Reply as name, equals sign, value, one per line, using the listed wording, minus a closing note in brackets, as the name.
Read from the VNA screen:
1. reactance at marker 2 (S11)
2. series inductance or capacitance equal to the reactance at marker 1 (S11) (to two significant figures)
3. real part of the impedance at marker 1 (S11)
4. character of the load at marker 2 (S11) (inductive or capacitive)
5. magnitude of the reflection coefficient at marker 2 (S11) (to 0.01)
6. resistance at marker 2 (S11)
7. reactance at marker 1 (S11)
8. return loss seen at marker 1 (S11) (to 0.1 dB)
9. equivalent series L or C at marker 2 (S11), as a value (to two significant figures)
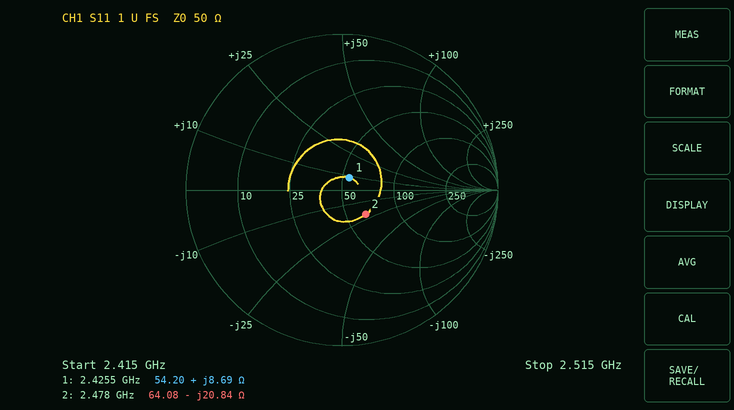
reactance at marker 2 = -20.84 Ω
series inductance or capacitance equal to the reactance at marker 1 (S11) = 570 pH
real part of the impedance at marker 1 = 54.20 Ω
character of the load at marker 2 (S11) = capacitive
magnitude of the reflection coefficient at marker 2 (S11) = 0.22
resistance at marker 2 = 64.08 Ω
reactance at marker 1 = +8.69 Ω
return loss seen at marker 1 (S11) = 20.7 dB
equivalent series L or C at marker 2 (S11), as a value = 3.1 pF
